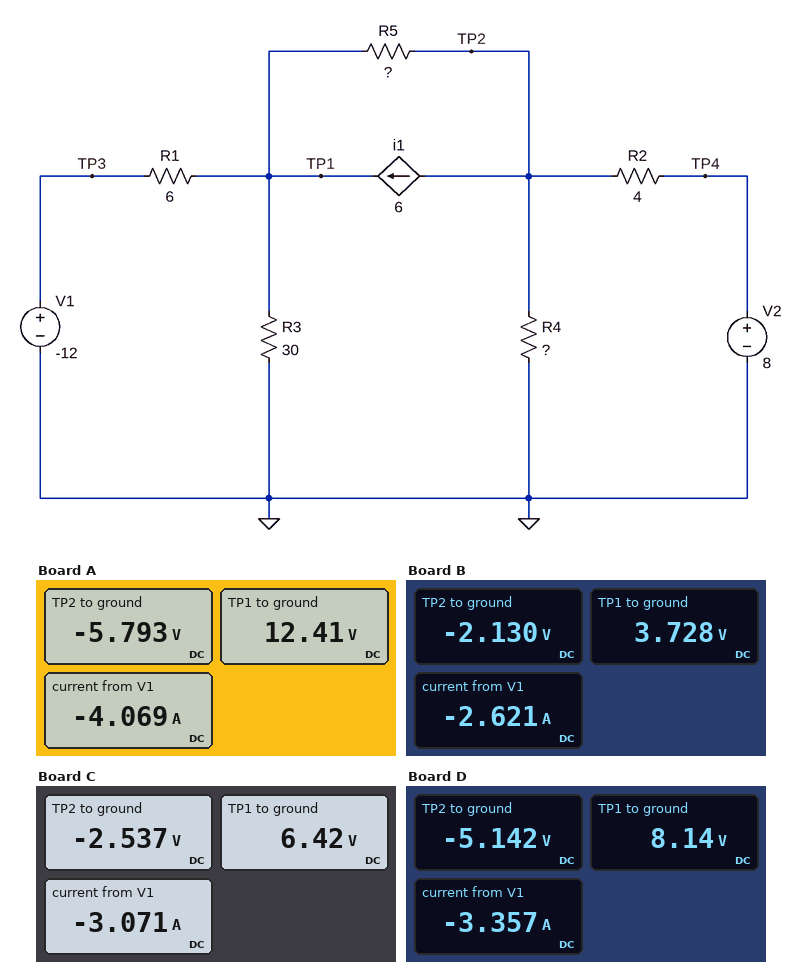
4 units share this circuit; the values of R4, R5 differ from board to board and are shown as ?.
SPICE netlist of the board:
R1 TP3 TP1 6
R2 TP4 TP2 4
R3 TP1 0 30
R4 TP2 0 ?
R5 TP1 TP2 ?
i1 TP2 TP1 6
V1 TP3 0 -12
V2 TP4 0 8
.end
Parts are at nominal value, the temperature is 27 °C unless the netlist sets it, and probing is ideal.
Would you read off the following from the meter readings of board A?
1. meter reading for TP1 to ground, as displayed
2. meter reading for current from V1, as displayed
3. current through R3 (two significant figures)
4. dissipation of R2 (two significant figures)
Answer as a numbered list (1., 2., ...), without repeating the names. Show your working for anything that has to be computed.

1. 12.41 V
2. -4.069 A
3. (12.41 V) / 30 Ω = 410 mA
4. (8 V - (-5.793 V))^2 / 4 Ω = 48 W
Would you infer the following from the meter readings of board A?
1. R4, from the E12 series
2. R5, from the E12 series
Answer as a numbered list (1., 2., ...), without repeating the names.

1. 5.6 Ω
2. 12 Ω
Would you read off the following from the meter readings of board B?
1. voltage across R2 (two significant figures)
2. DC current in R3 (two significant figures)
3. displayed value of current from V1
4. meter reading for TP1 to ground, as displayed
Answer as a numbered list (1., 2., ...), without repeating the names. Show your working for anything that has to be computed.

1. 8 V - (-2.13 V) = 10 V
2. (3.728 V) / 30 Ω = 120 mA
3. -2.621 A
4. 3.728 V
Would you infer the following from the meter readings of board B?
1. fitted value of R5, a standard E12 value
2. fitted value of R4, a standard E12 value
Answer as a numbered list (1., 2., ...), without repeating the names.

1. 1.8 Ω
2. 10 Ω
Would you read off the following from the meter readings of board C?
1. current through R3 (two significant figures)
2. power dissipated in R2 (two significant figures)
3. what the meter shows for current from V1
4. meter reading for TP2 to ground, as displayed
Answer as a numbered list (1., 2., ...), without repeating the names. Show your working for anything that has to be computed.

1. (6.42 V) / 30 Ω = 210 mA
2. (8 V - (-2.537 V))^2 / 4 Ω = 28 W
3. -3.071 A
4. -2.537 V
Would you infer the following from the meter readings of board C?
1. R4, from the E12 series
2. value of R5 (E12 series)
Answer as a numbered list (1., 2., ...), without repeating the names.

1. 3.9 Ω
2. 3.3 Ω
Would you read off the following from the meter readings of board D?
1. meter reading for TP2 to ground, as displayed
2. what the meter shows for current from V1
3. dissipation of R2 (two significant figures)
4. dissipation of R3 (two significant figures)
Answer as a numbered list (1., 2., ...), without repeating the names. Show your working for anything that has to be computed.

1. -5.142 V
2. -3.357 A
3. (8 V - (-5.142 V))^2 / 4 Ω = 43 W
4. (8.14 V)^2 / 30 Ω = 2.2 W
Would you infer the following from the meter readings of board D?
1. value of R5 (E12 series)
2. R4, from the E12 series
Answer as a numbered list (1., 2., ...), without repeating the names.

1. 5.6 Ω
2. 15 Ω
